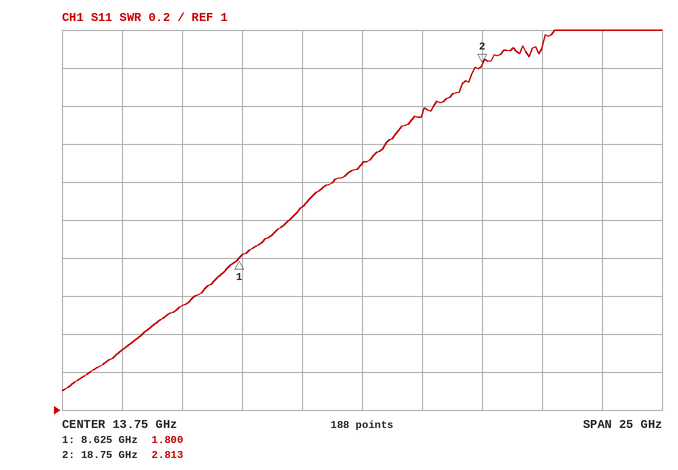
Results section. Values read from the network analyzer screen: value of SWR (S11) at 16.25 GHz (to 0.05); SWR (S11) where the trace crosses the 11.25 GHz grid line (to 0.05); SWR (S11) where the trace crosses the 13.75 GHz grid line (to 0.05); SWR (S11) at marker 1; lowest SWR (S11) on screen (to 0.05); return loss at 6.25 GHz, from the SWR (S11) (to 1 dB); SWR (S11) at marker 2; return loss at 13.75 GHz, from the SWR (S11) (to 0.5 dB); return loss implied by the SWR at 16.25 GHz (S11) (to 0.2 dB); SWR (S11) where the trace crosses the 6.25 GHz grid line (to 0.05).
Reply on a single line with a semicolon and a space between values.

2.55; 2.05; 2.30; 1.800; 1.10; 13 dB; 2.813; 8.0 dB; 7.2 dB; 1.55
